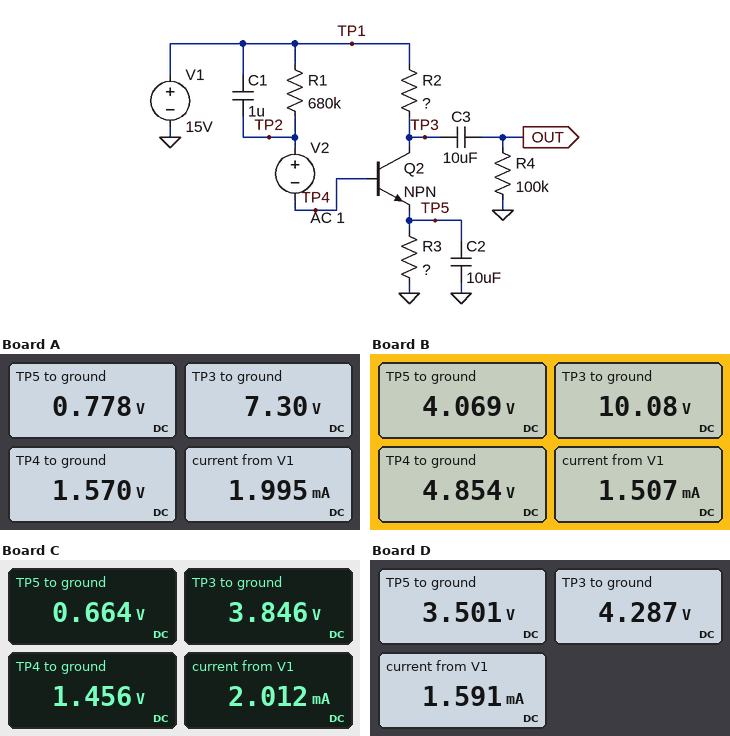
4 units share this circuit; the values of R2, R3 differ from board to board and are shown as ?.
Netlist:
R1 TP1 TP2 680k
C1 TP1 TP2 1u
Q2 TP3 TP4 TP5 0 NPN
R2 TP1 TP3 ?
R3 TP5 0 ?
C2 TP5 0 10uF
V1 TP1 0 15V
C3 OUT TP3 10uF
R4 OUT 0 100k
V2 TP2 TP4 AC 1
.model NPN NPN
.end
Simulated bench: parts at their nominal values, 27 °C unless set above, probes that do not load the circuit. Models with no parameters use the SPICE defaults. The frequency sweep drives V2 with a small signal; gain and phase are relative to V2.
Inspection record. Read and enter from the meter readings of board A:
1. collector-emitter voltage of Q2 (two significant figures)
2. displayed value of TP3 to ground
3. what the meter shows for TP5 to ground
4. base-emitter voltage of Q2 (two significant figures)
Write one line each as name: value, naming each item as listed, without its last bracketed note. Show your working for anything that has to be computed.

collector-emitter voltage of Q2: 7.3 V - 778 mV = 6.5 V
displayed value of TP3 to ground: 7.30 V
what the meter shows for TP5 to ground: 0.778 V
base-emitter voltage of Q2: 1.57 V - 778 mV = 790 mV
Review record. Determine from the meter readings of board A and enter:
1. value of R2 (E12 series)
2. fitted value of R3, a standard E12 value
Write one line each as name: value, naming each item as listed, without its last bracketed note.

value of R2: 3.9 kΩ
fitted value of R3, a standard E12 value: 390 Ω
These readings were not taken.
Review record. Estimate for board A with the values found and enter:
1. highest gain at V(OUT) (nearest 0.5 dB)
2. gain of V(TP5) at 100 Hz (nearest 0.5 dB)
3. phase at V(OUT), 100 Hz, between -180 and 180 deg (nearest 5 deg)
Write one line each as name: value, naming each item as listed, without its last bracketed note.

highest gain at V(OUT): 49.0 dB
gain of V(TP5) at 100 Hz: -1.0 dB
phase at V(OUT), 100 Hz, between -180 and 180 deg: 65 deg
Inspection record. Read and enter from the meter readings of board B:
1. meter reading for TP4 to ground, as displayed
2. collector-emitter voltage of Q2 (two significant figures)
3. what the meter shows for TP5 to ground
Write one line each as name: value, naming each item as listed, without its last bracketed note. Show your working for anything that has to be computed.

meter reading for TP4 to ground, as displayed: 4.854 V
collector-emitter voltage of Q2: 10.08 V - 4.069 V = 6.0 V
what the meter shows for TP5 to ground: 4.069 V
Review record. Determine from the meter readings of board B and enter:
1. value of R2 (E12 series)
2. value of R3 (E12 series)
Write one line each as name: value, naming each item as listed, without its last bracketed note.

value of R2: 3.3 kΩ
value of R3: 2.7 kΩ
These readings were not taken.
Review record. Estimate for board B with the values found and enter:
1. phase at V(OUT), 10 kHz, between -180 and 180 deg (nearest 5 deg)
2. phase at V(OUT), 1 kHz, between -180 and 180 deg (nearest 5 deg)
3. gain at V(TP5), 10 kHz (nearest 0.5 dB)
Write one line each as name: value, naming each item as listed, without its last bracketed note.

phase at V(OUT), 10 kHz, between -180 and 180 deg: 5 deg
phase at V(OUT), 1 kHz, between -180 and 180 deg: 45 deg
gain at V(TP5), 10 kHz: -20.5 dB
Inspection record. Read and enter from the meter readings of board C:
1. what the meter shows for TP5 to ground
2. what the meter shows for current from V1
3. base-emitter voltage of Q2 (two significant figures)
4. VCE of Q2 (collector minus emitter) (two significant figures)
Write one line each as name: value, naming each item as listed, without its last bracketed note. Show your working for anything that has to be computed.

what the meter shows for TP5 to ground: 0.664 V
what the meter shows for current from V1: 2.012 mA
base-emitter voltage of Q2: 1.456 V - 664 mV = 790 mV
VCE of Q2 (collector minus emitter): 3.846 V - 664 mV = 3.2 V
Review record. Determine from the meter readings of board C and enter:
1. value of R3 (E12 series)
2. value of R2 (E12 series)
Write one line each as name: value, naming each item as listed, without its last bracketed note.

value of R3: 330 Ω
value of R2: 5.6 kΩ
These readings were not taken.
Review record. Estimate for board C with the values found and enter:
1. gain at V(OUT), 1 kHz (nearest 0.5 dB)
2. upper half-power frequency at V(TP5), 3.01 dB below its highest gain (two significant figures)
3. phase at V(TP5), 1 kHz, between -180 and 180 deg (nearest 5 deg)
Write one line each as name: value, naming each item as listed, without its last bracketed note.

gain at V(OUT), 1 kHz: 47.5 dB
upper half-power frequency at V(TP5), 3.01 dB below its highest gain: 1.4 kHz
phase at V(TP5), 1 kHz, between -180 and 180 deg: 145 deg
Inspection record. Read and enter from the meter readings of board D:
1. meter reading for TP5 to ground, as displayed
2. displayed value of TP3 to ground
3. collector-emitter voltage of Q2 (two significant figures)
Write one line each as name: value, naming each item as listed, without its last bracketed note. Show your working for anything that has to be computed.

meter reading for TP5 to ground, as displayed: 3.501 V
displayed value of TP3 to ground: 4.287 V
collector-emitter voltage of Q2: 4.287 V - 3.501 V = 790 mV
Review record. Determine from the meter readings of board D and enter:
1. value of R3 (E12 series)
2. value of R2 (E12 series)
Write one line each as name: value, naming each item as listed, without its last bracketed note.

value of R3: 2.2 kΩ
value of R2: 6.8 kΩ
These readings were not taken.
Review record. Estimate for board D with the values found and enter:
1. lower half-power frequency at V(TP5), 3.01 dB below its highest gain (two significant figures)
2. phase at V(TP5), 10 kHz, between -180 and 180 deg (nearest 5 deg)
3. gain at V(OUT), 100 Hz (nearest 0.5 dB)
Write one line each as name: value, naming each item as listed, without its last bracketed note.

lower half-power frequency at V(TP5), 3.01 dB below its highest gain: 790 mHz
phase at V(TP5), 10 kHz, between -180 and 180 deg: 95 deg
gain at V(OUT), 100 Hz: 31.0 dB
